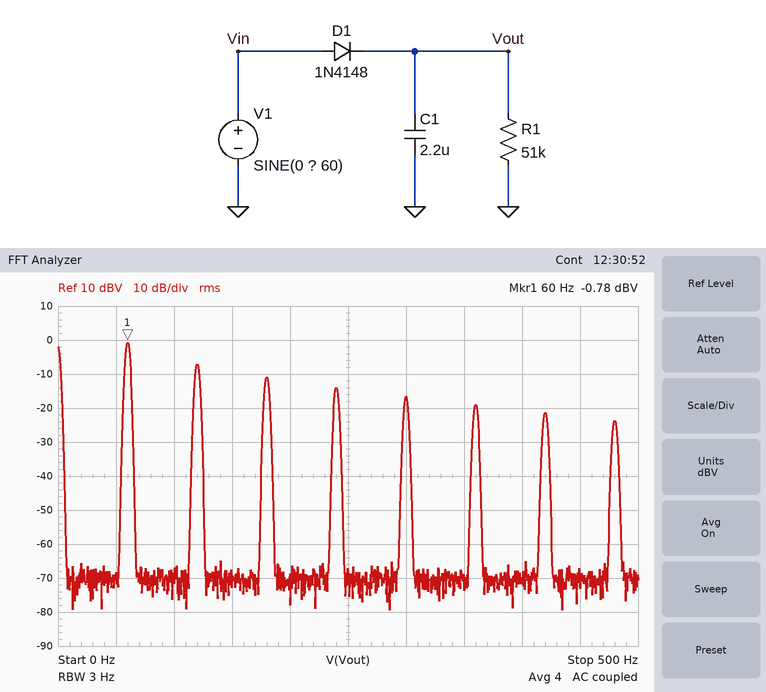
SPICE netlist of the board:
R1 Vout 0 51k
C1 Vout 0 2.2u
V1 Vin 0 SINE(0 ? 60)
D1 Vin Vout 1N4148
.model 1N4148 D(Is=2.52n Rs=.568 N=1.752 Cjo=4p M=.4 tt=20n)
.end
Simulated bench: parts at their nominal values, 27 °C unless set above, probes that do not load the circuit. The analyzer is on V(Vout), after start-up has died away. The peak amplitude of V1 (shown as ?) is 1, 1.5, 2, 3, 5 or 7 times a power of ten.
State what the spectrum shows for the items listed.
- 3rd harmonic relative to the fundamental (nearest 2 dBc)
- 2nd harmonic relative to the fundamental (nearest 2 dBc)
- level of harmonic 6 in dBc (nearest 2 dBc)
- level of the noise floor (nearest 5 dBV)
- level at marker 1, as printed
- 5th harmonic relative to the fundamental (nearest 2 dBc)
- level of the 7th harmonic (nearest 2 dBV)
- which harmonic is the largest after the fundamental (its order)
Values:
-10 dBc
-6 dBc
-18 dBc
-70 dBV
-0.78 dBV
-16 dBc
-22 dBV
2
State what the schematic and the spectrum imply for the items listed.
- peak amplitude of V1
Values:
30 V
